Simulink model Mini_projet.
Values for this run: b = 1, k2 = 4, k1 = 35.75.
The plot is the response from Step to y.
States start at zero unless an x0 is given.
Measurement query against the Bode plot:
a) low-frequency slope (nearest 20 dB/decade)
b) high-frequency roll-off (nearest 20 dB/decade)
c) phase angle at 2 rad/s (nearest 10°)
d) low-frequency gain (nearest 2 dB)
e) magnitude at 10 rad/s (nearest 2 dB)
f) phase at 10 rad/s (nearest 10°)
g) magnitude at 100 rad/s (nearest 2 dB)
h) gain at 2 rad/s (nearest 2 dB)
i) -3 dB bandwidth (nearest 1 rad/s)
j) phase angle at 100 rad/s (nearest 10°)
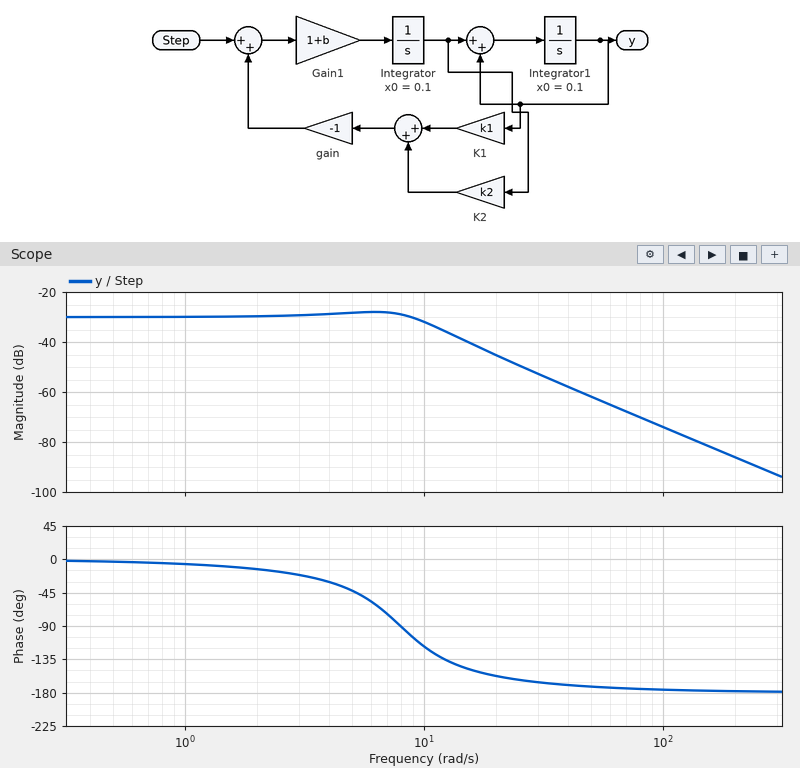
0 dB/decade
-40 dB/decade
-10°
-30 dB
-32 dB
-120°
-74 dB
-30 dB
11 rad/s
-180°
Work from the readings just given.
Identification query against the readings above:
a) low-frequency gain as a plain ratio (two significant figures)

0.032
